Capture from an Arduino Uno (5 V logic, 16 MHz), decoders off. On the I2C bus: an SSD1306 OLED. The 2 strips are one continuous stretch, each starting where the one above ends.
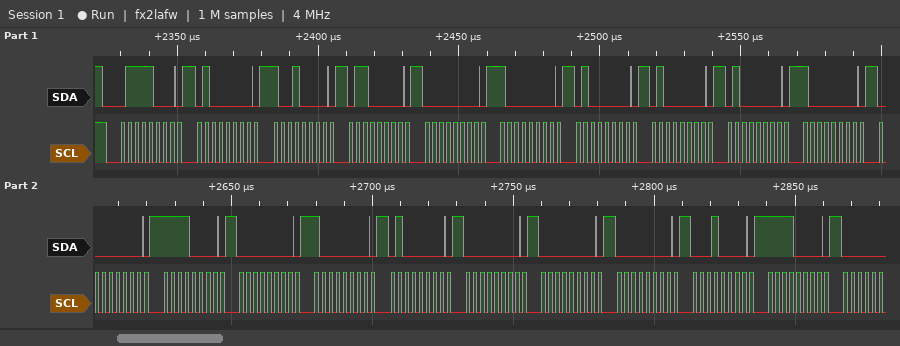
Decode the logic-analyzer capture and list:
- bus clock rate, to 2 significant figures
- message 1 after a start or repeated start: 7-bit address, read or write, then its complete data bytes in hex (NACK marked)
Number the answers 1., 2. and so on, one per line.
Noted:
1. 400 kHz
2. 0x3C write: 40 90 60 00 80 40 40 40 80 00 F0 00 80 40 00 00 00 10 F0
